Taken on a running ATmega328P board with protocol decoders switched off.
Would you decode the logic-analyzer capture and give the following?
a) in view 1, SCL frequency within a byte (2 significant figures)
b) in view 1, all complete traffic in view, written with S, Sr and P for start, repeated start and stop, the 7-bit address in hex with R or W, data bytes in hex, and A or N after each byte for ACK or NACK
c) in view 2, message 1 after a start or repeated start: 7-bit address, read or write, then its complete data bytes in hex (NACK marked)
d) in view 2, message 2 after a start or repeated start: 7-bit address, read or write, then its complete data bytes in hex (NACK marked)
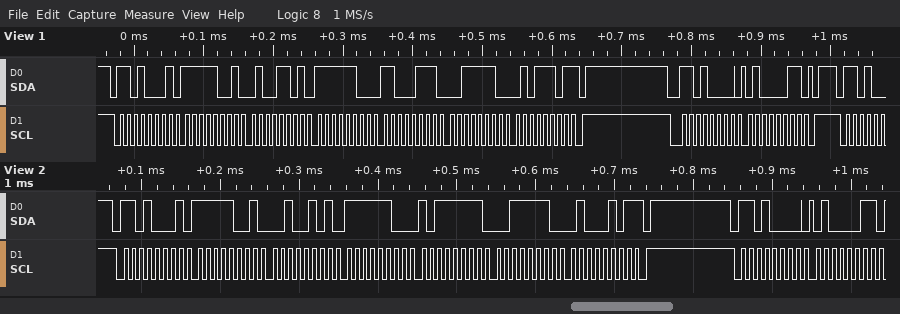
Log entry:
100 kHz
S 68R A F9 A 4D A FC A C7 A 3E A 5D N P S 68W A 43 A P
0x68 read: F9 25 FC BF 3E 45 NACK
0x68 write: 43
